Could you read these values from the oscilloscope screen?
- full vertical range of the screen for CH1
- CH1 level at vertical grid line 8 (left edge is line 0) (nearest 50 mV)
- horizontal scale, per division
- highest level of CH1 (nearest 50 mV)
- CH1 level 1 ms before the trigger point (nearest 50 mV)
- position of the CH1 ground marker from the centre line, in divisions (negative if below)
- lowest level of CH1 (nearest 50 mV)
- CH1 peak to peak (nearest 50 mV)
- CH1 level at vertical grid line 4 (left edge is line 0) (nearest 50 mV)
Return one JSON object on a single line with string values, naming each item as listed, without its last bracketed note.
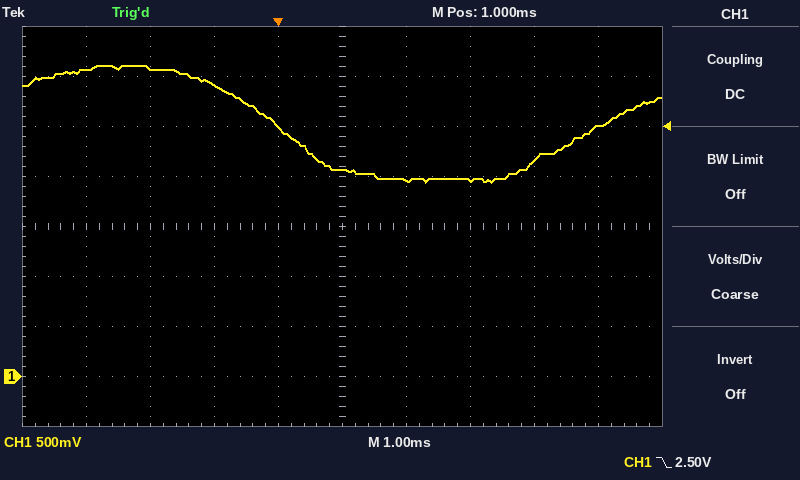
{"full vertical range of the screen for CH1": "4 V", "CH1 level at vertical grid line 8 (left edge is line 0)": "2.15 V", "horizontal scale, per division": "1 ms", "highest level of CH1": "3.10 V", "CH1 level 1 ms before the trigger point": "2.90 V", "position of the CH1 ground marker from the centre line, in divisions": "-3.0 div", "lowest level of CH1": "1.95 V", "CH1 peak to peak": "1.15 V", "CH1 level at vertical grid line 4 (left edge is line 0)": "2.50 V"}
